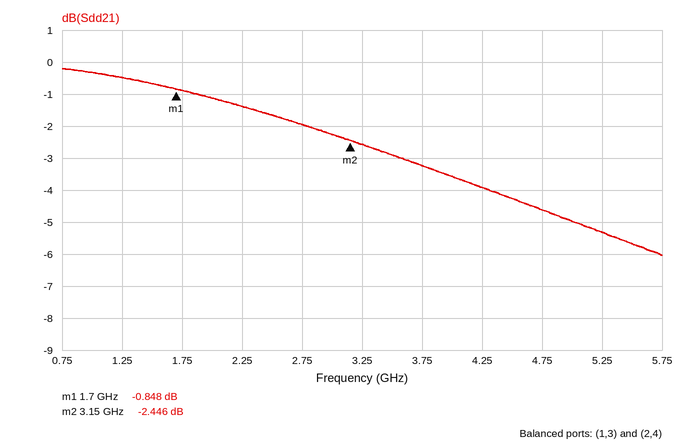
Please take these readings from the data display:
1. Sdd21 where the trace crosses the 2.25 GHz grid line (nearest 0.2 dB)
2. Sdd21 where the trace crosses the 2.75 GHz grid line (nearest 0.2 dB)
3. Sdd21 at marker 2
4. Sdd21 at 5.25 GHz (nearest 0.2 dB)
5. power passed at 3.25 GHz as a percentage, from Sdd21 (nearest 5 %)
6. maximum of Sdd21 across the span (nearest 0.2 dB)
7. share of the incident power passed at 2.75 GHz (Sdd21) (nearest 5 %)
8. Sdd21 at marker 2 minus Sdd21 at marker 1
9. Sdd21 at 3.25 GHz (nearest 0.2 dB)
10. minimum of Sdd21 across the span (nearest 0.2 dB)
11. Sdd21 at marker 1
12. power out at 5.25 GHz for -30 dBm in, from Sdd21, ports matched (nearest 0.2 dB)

-1.4 dB
-2.0 dB
-2.446 dB
-5.4 dB
55 %
-0.2 dB
65 %
-1.598 dB
-2.6 dB
-6.0 dB
-0.848 dB
-35.4 dBm
